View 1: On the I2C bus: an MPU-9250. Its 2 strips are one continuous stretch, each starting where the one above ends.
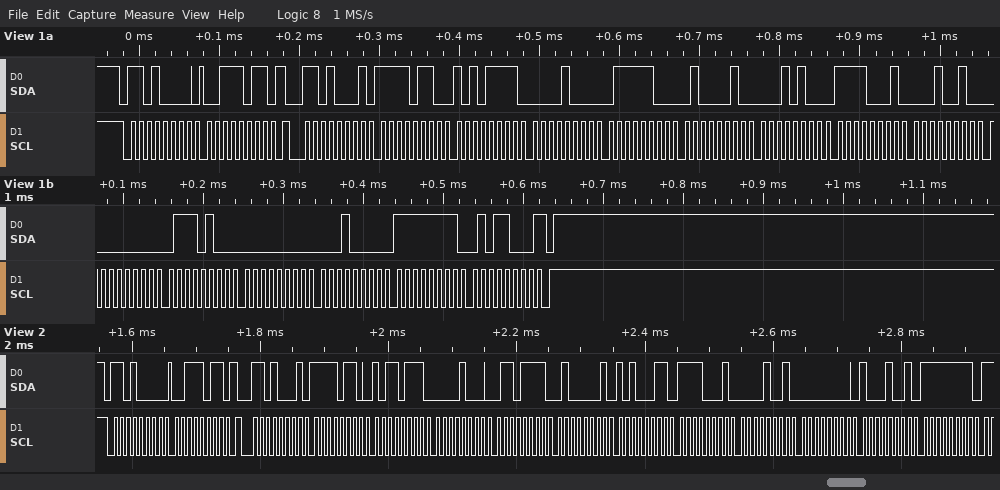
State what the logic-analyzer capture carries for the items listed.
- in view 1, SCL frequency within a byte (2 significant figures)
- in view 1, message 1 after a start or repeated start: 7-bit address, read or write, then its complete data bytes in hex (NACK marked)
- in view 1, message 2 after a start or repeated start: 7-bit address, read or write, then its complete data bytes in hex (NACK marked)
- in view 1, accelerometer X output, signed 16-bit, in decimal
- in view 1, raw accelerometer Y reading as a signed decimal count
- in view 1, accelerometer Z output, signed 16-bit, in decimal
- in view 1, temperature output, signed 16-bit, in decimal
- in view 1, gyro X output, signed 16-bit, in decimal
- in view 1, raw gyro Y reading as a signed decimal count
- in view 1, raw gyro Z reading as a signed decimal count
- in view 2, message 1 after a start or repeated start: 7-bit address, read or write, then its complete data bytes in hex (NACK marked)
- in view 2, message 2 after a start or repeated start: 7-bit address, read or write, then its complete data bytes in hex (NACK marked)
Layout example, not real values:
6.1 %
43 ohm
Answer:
100 kHz
0x68 write: 3B
0x68 read: F6 AF 08 7C 42 14 F1 12 00 74 00 10 FF 58 NACK
-2385
2172
16916
-3822
116
16
-168
0x68 write: 3B
0x68 read: F6 B7 08 6F 41 A3 F1 09 00 89 FF
